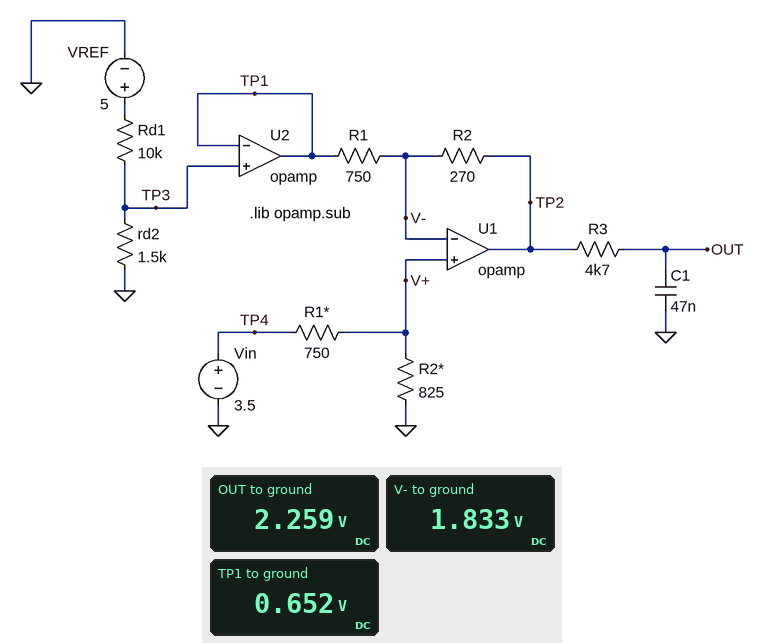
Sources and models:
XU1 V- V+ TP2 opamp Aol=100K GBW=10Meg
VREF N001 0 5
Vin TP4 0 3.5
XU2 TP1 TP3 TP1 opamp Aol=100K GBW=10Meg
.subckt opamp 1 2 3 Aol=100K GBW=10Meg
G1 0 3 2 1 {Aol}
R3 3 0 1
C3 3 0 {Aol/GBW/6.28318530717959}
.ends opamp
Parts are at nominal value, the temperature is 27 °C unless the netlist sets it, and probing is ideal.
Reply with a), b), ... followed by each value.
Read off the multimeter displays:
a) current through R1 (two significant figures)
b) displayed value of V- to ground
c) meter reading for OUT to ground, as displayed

a) 1.6 mA
b) 1.833 V
c) 2.259 V
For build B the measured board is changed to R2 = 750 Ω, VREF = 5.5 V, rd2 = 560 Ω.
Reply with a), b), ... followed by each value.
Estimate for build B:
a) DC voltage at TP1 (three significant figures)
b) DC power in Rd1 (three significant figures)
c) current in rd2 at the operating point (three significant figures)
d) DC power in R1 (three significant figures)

a) 292 mV
b) 2.71 mW
c) 521 µA
d) 3.17 mW
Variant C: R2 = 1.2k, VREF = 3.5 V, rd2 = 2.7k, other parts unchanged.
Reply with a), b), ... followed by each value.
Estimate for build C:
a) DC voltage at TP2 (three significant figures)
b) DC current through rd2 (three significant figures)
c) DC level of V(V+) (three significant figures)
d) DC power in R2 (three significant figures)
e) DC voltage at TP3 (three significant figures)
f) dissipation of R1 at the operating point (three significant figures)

a) 3.58 V
b) 276 µA
c) 1.83 V
d) 2.53 mW
e) 744 mV
f) 1.58 mW
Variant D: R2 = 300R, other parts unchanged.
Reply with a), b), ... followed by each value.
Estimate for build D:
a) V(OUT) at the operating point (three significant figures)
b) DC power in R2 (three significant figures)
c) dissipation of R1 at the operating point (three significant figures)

a) 2.31 V
b) 744 µW
c) 1.86 mW
